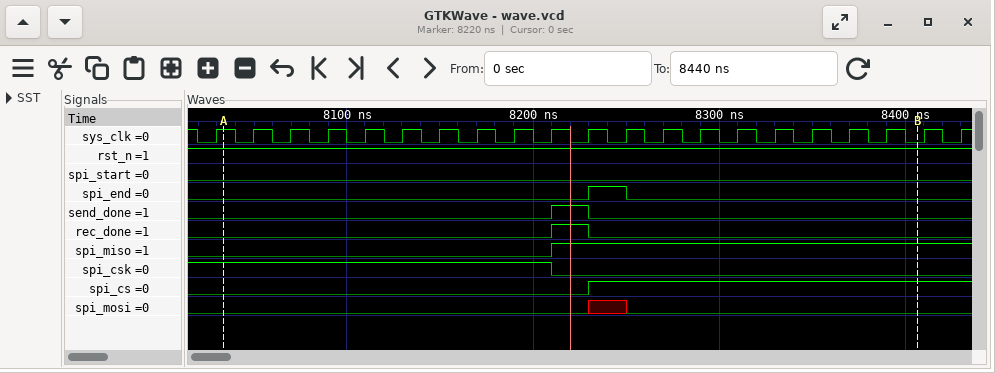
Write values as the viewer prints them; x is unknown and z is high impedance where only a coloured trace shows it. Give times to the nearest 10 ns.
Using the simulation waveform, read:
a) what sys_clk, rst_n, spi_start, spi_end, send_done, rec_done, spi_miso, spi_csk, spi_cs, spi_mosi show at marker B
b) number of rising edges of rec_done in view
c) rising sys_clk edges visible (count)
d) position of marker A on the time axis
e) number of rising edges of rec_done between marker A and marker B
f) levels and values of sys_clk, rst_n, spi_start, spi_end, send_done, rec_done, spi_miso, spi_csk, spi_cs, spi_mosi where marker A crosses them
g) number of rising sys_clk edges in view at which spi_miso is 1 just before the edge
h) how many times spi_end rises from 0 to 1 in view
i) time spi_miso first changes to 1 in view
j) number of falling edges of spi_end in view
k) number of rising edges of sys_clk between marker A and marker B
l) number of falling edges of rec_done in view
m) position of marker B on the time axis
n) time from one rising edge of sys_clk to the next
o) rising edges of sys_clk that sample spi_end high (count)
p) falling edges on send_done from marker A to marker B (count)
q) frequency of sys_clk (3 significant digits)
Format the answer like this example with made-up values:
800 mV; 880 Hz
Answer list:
sys_clk=0, rst_n=1, spi_start=0, spi_end=0, send_done=0, rec_done=0, spi_miso=1, spi_csk=0, spi_cs=1, spi_mosi=0; 1; 21; 8030 ns; 1; sys_clk=1, rst_n=1, spi_start=0, spi_end=0, send_done=0, rec_done=0, spi_miso=0, spi_csk=1, spi_cs=0, spi_mosi=0; 11; 1; 8210 ns; 1; 18; 1; 8410 ns; 20 ns; 1; 1; 50.0 MHz
